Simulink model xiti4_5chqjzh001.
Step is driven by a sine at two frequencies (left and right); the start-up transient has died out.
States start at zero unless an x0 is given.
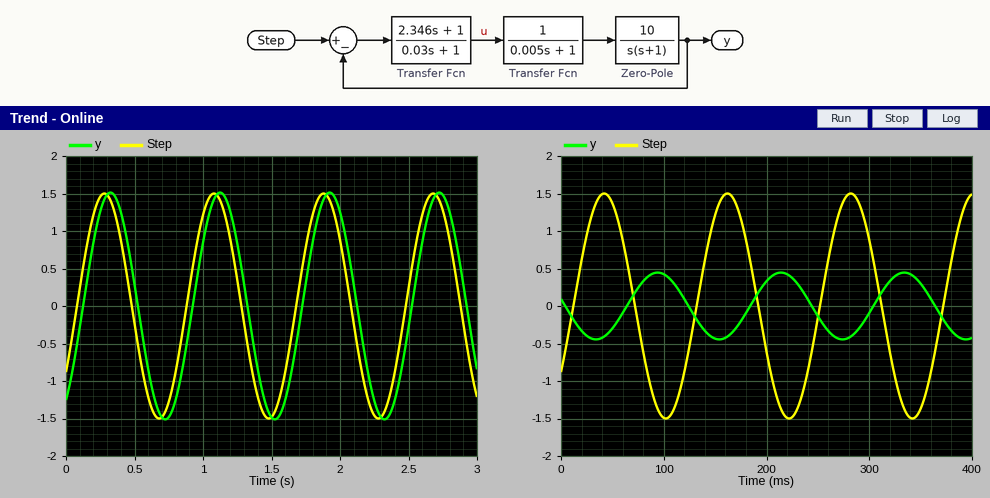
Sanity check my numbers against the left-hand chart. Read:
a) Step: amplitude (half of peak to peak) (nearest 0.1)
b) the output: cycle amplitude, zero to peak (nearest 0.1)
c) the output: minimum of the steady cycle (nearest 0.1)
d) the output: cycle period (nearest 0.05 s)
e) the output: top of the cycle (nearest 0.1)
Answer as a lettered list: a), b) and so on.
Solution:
a) 1.5
b) 1.5
c) -1.5
d) 0.80 s
e) 1.5
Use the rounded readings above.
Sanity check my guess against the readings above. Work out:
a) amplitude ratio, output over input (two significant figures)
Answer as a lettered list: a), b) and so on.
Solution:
a) 1.0
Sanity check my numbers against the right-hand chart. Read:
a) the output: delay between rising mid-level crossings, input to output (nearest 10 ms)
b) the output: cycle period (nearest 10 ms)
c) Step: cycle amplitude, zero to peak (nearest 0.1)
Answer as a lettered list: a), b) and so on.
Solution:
a) 50 ms
b) 120 ms
c) 1.5
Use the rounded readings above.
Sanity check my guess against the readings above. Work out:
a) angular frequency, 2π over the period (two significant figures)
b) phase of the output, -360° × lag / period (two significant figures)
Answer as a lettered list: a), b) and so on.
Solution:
a) 0.052 rad/ms
b) -150°
